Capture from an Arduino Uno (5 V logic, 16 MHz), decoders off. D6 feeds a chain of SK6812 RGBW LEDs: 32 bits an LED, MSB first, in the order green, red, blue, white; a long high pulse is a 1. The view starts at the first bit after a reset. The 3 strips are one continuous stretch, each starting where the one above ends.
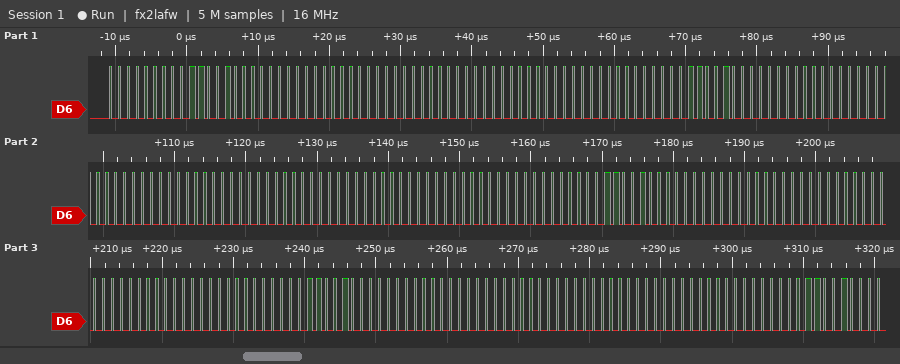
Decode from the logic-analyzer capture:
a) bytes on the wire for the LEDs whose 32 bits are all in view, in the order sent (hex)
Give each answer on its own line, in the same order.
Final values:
00 64 00 00 00 00 00 00 64 00 00 00 00 00 00 00 00 00 64 00 00 00 00 00 00 64 00 00 00 00 00 00
